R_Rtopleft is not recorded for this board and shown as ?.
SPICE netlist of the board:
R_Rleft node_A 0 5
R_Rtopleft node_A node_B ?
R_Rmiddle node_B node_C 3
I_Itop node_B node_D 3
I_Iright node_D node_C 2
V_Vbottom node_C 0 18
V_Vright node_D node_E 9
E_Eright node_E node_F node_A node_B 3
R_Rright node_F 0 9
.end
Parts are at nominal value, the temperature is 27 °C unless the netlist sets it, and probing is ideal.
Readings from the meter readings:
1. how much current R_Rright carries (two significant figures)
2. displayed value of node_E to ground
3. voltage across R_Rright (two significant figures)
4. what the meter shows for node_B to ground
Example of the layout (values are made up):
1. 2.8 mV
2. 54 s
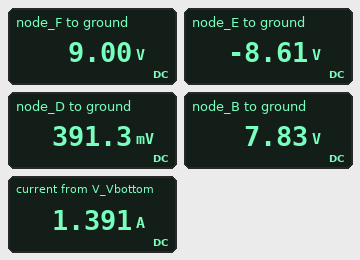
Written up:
1. 1.0 A
2. -8.61 V
3. 9.0 V
4. 7.83 V
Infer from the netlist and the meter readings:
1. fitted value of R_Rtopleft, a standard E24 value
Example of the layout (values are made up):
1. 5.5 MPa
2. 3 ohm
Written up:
1. 15 Ω
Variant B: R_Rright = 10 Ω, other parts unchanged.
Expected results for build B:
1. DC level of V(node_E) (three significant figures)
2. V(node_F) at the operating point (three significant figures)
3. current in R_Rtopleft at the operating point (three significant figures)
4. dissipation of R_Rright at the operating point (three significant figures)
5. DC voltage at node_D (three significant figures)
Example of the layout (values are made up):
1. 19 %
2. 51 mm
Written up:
1. -7.61 V
2. 10.0 V
3. 391 mA
4. 10.0 W
5. 1.39 V
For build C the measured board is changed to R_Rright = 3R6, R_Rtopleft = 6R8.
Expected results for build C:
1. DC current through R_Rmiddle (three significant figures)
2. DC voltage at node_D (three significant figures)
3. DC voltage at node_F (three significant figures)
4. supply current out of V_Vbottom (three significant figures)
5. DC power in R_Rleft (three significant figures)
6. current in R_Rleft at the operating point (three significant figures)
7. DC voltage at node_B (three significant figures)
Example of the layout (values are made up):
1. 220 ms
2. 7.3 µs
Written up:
1. 3.61 A
2. 195 mV
3. 3.60 V
4. 1.61 A
5. 1.85 W
6. 608 mA
7. 7.18 V
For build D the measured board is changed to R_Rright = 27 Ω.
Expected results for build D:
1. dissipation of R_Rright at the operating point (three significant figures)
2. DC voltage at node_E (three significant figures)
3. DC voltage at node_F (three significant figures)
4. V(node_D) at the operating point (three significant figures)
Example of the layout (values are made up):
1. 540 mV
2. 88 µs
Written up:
1. 27.0 W
2. 9.39 V
3. 27.0 V
4. 18.4 V
